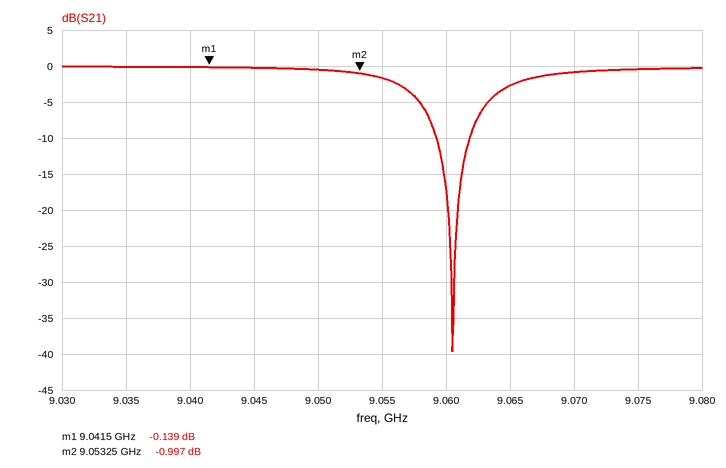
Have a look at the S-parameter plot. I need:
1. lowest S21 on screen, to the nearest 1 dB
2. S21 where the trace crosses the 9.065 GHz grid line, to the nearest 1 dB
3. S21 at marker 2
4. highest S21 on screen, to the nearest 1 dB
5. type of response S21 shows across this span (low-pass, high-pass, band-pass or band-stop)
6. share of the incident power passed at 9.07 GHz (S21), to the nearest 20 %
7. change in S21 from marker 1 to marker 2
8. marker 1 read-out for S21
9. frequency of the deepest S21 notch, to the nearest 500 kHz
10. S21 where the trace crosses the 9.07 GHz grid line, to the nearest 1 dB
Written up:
-40 dB
-3 dB
-0.997 dB
0 dB
band-stop
80 %
-0.858 dB
-0.139 dB
9.0605 GHz
-1 dB
